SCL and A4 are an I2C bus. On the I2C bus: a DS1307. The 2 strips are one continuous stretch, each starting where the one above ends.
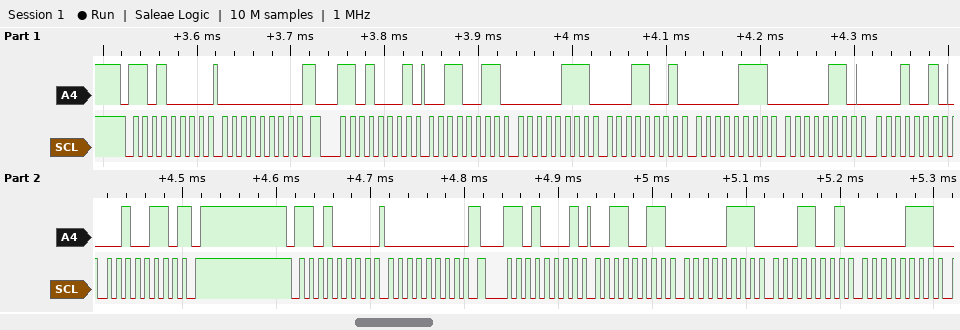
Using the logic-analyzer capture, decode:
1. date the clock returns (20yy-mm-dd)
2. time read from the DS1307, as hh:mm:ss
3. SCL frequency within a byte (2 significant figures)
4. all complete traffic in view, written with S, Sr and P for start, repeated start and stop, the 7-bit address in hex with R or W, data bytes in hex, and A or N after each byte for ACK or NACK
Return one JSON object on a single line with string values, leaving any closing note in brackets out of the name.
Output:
{"date the clock returns": "2026-12-06", "time read from the DS1307, as hh:mm:ss": "19:07:33", "SCL frequency within a byte": "100 kHz", "all complete traffic in view, written with S, Sr and P for start, repeated start and stop, the 7-bit address in hex with R or W, data bytes in hex, and A or N after each byte for ACK or NACK": "S 68W A 00 A Sr 68R A 33 A 07 A 19 A 07 A 06 A 12 A 26 N P S 68W A 00 A Sr 68R A 33 A 07 A 19 A 07 A"}
